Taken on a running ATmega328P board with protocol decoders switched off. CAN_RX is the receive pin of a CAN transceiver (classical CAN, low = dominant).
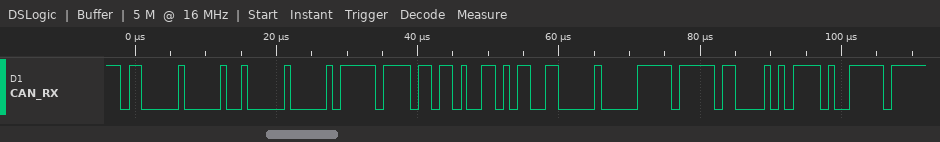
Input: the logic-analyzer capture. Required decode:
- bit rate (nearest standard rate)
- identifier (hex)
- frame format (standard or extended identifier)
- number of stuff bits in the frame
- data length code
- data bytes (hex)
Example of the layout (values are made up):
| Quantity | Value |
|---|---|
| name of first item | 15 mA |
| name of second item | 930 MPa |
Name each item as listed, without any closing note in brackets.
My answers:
| Quantity | Value |
|---|---|
| bit rate | 1000 kbit/s |
| identifier | 0x600 |
| frame format | standard |
| number of stuff bits in the frame | 9 |
| data length code | 8 |
| data bytes | 00 FF B6 9A CC 00 FF E1 |
